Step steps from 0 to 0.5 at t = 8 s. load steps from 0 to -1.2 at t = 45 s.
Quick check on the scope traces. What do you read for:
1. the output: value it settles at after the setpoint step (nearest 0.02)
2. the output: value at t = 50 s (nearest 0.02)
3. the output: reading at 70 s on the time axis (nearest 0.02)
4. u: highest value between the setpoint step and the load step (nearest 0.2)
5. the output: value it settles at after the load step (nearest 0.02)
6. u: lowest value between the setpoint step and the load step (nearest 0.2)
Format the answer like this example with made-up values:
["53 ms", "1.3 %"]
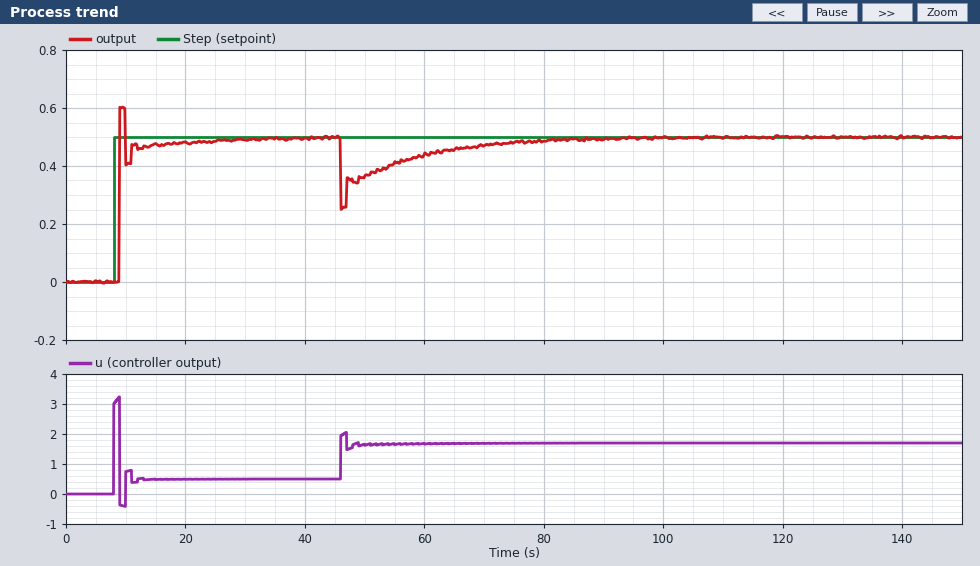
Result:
["0.50", "0.36", "0.48", "3.2", "0.50", "-0.4"]
